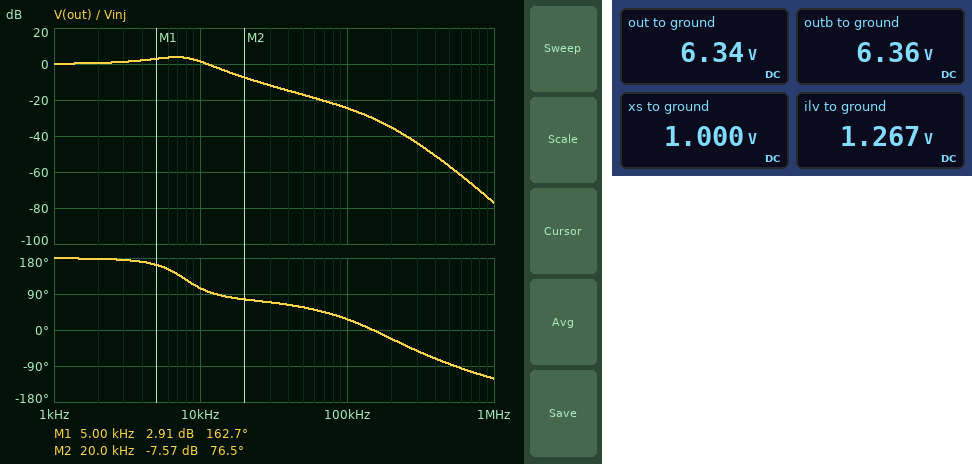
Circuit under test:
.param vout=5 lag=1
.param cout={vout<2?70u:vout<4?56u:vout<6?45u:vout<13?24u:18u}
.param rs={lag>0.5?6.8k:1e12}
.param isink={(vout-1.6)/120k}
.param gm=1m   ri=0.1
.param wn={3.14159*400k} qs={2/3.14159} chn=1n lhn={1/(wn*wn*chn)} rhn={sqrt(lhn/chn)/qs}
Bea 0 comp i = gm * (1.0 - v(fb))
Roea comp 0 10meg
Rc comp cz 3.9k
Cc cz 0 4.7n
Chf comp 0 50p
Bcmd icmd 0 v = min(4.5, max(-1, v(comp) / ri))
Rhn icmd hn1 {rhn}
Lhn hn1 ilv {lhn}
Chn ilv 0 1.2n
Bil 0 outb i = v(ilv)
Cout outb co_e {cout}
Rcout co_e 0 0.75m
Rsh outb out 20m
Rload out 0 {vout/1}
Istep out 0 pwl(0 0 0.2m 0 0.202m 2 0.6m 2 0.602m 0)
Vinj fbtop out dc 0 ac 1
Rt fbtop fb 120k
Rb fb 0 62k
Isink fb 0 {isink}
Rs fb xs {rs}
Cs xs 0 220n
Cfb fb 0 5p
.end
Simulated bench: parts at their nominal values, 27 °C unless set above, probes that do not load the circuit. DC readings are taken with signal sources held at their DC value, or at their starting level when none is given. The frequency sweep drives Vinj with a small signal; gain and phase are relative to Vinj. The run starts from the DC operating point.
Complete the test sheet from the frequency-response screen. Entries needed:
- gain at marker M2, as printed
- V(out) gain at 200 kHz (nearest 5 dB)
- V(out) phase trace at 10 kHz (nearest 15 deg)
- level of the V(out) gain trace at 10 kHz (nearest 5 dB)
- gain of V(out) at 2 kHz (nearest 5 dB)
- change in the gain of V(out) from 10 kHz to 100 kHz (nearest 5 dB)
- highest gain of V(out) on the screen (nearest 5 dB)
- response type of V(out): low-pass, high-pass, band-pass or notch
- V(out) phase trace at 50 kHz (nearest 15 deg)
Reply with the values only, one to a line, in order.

-7.57 dB
-35 dB
105 deg
0 dB
0 dB
-25 dB
5 dB
low-pass
60 deg
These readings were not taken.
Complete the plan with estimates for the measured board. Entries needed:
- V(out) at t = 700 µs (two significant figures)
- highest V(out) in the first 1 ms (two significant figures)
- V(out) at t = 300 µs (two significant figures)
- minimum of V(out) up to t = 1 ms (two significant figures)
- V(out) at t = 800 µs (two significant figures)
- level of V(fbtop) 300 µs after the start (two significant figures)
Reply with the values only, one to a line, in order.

6.2 V
6.9 V
6.5 V
5.8 V
6.3 V
6.5 V
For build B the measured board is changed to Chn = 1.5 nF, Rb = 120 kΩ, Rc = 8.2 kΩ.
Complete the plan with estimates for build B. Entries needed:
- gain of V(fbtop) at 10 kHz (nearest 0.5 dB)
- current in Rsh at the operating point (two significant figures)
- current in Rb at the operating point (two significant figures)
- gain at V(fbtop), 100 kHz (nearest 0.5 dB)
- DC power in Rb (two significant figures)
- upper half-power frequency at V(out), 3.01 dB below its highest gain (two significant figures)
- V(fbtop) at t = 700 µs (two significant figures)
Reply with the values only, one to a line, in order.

-3.0 dB
1.1 A
8.3 µA
1.0 dB
8.3 µW
18 kHz
5.4 V
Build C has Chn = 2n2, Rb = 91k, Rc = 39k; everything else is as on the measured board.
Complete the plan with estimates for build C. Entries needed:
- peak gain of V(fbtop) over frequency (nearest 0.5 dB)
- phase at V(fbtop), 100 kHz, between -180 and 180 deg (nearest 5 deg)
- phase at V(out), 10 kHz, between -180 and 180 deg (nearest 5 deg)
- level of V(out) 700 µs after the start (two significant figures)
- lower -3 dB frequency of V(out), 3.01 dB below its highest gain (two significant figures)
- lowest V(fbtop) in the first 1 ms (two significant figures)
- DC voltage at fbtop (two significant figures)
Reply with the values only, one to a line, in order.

13.5 dB
-10 deg
170 deg
5.8 V
45 kHz
5.5 V
5.7 V
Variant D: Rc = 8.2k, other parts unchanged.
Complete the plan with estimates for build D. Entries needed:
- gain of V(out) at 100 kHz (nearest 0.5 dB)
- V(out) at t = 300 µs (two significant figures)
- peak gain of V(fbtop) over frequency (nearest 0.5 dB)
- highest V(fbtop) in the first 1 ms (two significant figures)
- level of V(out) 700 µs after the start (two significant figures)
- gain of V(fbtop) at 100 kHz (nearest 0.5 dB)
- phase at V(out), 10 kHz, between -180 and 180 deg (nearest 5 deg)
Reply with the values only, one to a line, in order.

-18.0 dB
6.3 V
1.5 dB
6.7 V
6.4 V
1.0 dB
140 deg
